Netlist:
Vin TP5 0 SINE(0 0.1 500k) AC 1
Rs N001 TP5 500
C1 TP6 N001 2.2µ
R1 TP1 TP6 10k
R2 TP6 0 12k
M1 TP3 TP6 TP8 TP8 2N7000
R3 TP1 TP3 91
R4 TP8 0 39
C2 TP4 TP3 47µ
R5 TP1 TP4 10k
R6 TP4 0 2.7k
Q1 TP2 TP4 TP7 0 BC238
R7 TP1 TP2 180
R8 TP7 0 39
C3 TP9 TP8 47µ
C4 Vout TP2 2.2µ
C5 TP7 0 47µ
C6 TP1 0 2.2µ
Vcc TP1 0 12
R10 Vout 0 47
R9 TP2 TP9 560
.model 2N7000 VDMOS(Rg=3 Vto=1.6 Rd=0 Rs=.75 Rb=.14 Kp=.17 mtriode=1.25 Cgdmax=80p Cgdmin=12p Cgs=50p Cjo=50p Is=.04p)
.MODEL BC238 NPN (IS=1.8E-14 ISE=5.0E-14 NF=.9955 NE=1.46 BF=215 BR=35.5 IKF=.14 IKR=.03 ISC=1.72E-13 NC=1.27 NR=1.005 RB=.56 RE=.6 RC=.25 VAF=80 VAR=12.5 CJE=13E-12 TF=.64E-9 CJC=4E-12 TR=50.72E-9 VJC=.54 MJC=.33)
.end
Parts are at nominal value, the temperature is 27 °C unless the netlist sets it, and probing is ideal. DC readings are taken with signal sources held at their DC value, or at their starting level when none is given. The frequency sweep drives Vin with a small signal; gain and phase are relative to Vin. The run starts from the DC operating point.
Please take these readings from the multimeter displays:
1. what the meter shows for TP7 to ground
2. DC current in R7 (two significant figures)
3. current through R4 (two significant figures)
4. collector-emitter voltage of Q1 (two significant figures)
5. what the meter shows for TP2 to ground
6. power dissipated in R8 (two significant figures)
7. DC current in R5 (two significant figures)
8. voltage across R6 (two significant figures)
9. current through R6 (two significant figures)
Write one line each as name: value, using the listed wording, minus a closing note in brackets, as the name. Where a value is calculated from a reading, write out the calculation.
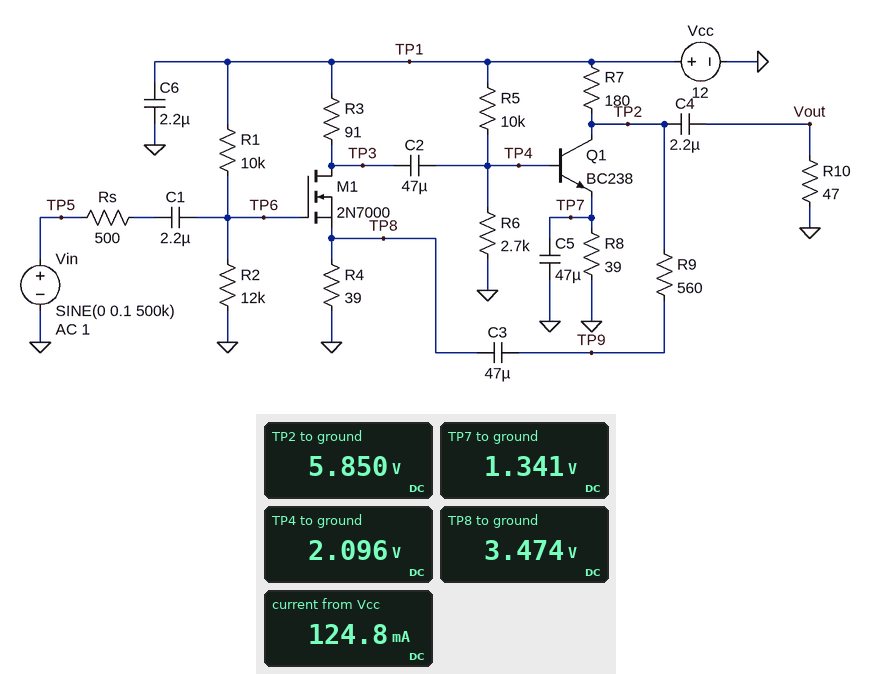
what the meter shows for TP7 to ground: 1.341 V
DC current in R7: (12 V - 5.85 V) / 180 Ω = 34 mA
current through R4: (3.474 V) / 39 Ω = 89 mA
collector-emitter voltage of Q1: 5.85 V - 1.341 V = 4.5 V
what the meter shows for TP2 to ground: 5.850 V
power dissipated in R8: (1.341 V)^2 / 39 Ω = 46 mW
DC current in R5: (12 V - 2.096 V) / 10 kΩ = 990 µA
voltage across R6: 2.096 V = 2.1 V
current through R6: (2.096 V) / 2.7 kΩ = 780 µA
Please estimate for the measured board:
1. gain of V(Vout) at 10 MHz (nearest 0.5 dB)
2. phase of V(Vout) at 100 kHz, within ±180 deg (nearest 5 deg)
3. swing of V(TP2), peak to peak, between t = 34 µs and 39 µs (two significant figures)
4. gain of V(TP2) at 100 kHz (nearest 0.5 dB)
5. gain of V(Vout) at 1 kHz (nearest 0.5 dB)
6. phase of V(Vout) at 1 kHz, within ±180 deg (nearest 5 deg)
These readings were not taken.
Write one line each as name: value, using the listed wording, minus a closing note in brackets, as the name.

gain of V(Vout) at 10 MHz: -3.5 dB
phase of V(Vout) at 100 kHz, within ±180 deg: 0 deg
swing of V(TP2), peak to peak, between t = 34 µs and 39 µs: 390 mV
gain of V(TP2) at 100 kHz: 6.0 dB
gain of V(Vout) at 1 kHz: -0.5 dB
phase of V(Vout) at 1 kHz, within ±180 deg: 70 deg
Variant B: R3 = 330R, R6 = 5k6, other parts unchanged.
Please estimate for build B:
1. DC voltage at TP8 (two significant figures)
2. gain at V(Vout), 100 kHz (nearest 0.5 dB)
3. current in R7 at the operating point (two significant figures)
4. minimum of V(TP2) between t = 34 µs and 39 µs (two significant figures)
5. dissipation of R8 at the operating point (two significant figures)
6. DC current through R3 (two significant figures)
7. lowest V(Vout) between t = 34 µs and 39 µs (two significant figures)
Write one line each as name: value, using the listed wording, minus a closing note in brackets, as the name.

DC voltage at TP8: 1.3 V
gain at V(Vout), 100 kHz: -20.5 dB
current in R7 at the operating point: 53 mA
minimum of V(TP2) between t = 34 µs and 39 µs: 2.4 V
dissipation of R8 at the operating point: 110 mW
DC current through R3: 32 mA
lowest V(Vout) between t = 34 µs and 39 µs: -15 mV
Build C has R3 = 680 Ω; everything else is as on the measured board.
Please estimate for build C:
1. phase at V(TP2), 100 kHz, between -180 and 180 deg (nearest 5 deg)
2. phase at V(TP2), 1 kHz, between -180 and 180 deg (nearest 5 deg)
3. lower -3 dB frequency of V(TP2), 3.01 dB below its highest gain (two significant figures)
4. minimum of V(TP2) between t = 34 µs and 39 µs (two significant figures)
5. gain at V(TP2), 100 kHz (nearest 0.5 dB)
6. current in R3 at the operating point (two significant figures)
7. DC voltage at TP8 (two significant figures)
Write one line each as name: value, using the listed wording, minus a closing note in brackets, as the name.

phase at V(TP2), 100 kHz, between -180 and 180 deg: -40 deg
phase at V(TP2), 1 kHz, between -180 and 180 deg: 10 deg
lower -3 dB frequency of V(TP2), 3.01 dB below its highest gain: 2.1 MHz
minimum of V(TP2) between t = 34 µs and 39 µs: 5.8 V
gain at V(TP2), 100 kHz: -28.0 dB
current in R3 at the operating point: 17 mA
DC voltage at TP8: 650 mV
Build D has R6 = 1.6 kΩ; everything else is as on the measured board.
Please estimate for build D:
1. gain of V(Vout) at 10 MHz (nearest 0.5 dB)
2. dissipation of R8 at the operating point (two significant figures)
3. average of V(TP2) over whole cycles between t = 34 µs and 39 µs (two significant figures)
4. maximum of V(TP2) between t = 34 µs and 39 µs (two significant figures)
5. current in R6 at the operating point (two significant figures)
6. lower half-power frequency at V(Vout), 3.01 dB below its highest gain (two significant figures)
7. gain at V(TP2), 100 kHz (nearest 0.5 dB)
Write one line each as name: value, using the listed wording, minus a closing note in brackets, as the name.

gain of V(Vout) at 10 MHz: -4.5 dB
dissipation of R8 at the operating point: 15 mW
average of V(TP2) over whole cycles between t = 34 µs and 39 µs: 8.4 V
maximum of V(TP2) between t = 34 µs and 39 µs: 8.6 V
current in R6 at the operating point: 940 µA
lower half-power frequency at V(Vout), 3.01 dB below its highest gain: 1.6 kHz
gain at V(TP2), 100 kHz: 4.5 dB
